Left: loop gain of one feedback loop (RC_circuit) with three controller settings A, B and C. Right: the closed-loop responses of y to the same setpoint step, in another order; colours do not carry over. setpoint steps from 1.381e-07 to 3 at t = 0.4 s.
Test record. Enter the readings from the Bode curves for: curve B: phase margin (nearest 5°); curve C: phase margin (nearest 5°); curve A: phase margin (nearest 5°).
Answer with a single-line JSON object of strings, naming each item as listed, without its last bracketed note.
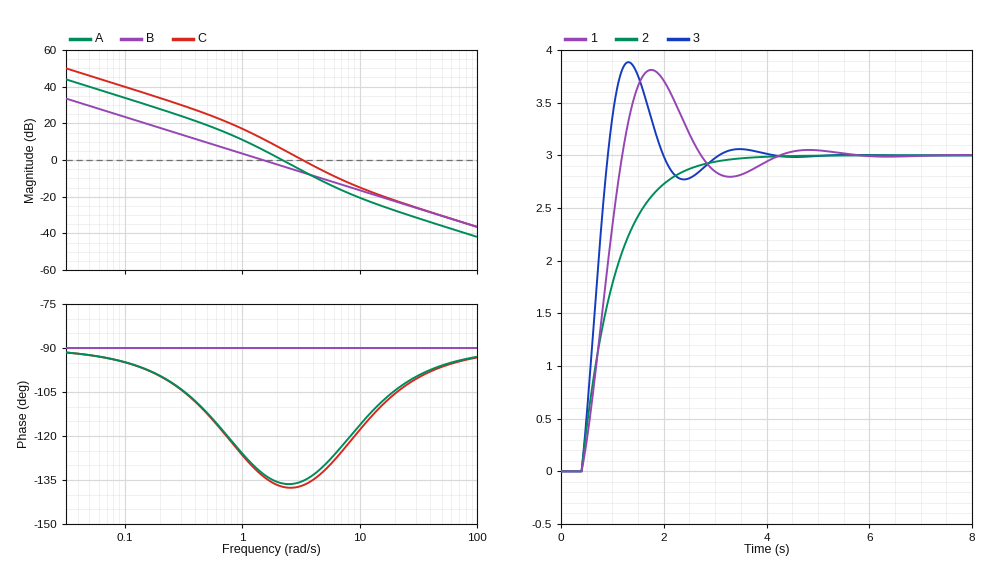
{"curve B: phase margin": "90°", "curve C: phase margin": "45°", "curve A: phase margin": "45°"}
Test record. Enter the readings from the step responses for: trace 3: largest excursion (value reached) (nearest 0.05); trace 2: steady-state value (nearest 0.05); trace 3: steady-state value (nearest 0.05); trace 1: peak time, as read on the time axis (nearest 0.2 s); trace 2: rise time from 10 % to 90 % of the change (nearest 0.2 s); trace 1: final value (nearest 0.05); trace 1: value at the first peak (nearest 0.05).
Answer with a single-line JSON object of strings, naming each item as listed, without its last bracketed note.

{"trace 3: largest excursion (value reached)": "3.90", "trace 2: steady-state value": "3.00", "trace 3: steady-state value": "3.00", "trace 1: peak time, as read on the time axis": "1.8 s", "trace 2: rise time from 10 % to 90 % of the change": "1.4 s", "trace 1: final value": "3.00", "trace 1: value at the first peak": "3.80"}
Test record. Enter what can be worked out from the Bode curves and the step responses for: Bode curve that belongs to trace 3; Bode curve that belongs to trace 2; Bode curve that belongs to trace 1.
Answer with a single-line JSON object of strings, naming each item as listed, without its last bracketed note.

{"Bode curve that belongs to trace 3": "C", "Bode curve that belongs to trace 2": "B", "Bode curve that belongs to trace 1": "A"}
